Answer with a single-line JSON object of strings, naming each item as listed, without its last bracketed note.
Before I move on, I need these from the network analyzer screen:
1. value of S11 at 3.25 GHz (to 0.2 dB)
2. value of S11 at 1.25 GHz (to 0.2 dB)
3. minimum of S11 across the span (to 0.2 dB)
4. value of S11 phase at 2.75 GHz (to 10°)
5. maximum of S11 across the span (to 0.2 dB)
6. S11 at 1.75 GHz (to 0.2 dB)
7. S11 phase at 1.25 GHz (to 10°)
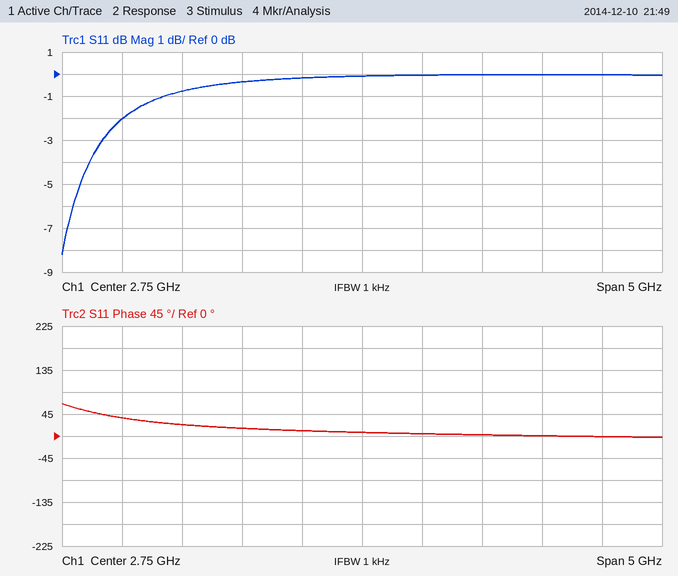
{"value of S11 at 3.25 GHz": "0.0 dB", "value of S11 at 1.25 GHz": "-0.8 dB", "minimum of S11 across the span": "-8.2 dB", "value of S11 phase at 2.75 GHz": "10°", "maximum of S11 across the span": "0.0 dB", "S11 at 1.75 GHz": "-0.4 dB", "S11 phase at 1.25 GHz": "20°"}
